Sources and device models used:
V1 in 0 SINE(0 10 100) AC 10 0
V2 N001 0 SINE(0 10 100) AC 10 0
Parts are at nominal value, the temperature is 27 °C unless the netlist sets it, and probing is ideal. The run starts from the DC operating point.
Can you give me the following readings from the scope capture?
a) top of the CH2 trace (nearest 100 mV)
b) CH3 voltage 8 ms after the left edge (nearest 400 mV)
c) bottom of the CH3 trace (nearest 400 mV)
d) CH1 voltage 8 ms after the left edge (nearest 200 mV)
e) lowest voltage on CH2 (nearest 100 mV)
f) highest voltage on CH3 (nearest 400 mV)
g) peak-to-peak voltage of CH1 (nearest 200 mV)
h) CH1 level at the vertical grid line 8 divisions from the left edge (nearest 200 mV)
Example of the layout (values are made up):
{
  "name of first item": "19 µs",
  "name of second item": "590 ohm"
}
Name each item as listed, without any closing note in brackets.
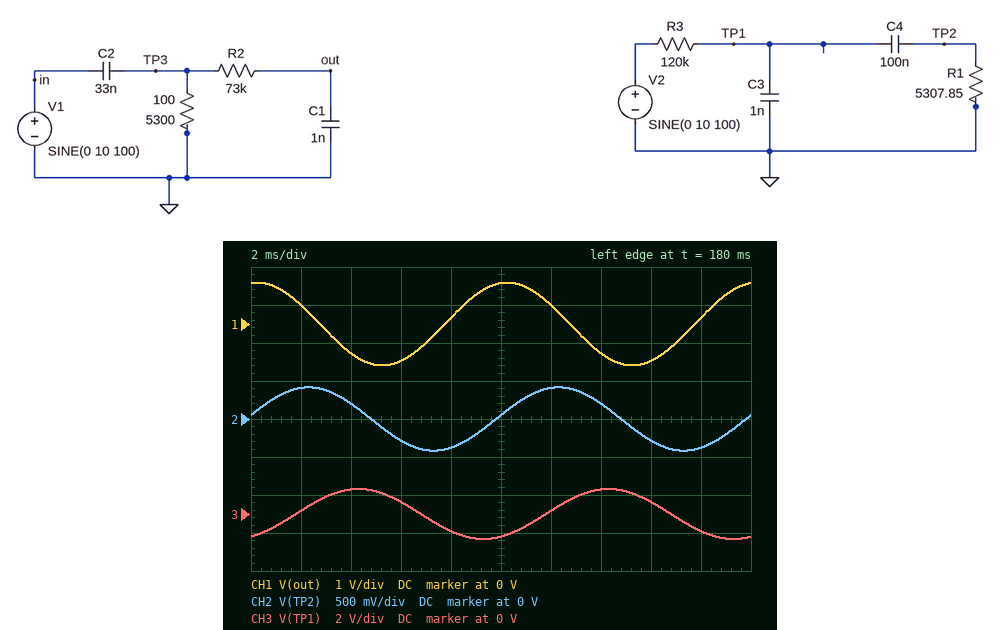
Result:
{
  "top of the CH2 trace": "400 mV",
  "CH3 voltage 8 ms after the left edge": "-800 mV",
  "bottom of the CH3 trace": "-1.2 V",
  "CH1 voltage 8 ms after the left edge": "200 mV",
  "lowest voltage on CH2": "-400 mV",
  "highest voltage on CH3": "1.2 V",
  "peak-to-peak voltage of CH1": "2.2 V",
  "CH1 level at the vertical grid line 8 divisions from the left edge": "-1.0 V"
}
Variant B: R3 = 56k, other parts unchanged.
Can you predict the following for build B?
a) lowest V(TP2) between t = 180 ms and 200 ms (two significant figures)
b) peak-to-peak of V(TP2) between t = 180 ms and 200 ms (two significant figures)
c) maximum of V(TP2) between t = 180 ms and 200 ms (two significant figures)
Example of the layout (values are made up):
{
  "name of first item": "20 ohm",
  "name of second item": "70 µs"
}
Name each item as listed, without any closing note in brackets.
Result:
{
  "lowest V(TP2) between t = 180 ms and 200 ms": "-830 mV",
  "peak-to-peak of V(TP2) between t = 180 ms and 200 ms": "1.7 V",
  "maximum of V(TP2) between t = 180 ms and 200 ms": "830 mV"
}
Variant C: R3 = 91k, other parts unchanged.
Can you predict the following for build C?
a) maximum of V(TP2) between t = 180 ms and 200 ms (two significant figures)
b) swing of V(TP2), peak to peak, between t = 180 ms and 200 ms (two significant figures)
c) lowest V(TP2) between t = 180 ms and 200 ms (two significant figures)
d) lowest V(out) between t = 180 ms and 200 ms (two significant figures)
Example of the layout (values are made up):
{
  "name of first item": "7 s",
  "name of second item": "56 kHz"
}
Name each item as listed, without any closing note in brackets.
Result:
{
  "maximum of V(TP2) between t = 180 ms and 200 ms": "540 mV",
  "swing of V(TP2), peak to peak, between t = 180 ms and 200 ms": "1.1 V",
  "lowest V(TP2) between t = 180 ms and 200 ms": "-540 mV",
  "lowest V(out) between t = 180 ms and 200 ms": "-1.1 V"
}
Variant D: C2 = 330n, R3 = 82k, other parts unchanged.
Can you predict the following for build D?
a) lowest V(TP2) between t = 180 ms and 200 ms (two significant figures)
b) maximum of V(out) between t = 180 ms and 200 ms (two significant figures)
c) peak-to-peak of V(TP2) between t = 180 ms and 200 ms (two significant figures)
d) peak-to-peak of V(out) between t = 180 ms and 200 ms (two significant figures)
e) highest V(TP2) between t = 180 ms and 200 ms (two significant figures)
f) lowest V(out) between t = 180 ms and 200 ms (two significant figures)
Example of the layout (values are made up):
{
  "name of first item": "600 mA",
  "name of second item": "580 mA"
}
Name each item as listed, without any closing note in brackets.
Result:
{
  "lowest V(TP2) between t = 180 ms and 200 ms": "-590 mV",
  "maximum of V(out) between t = 180 ms and 200 ms": "7.4 V",
  "peak-to-peak of V(TP2) between t = 180 ms and 200 ms": "1.2 V",
  "peak-to-peak of V(out) between t = 180 ms and 200 ms": "15 V",
  "highest V(TP2) between t = 180 ms and 200 ms": "590 mV",
  "lowest V(out) between t = 180 ms and 200 ms": "-7.4 V"
}
